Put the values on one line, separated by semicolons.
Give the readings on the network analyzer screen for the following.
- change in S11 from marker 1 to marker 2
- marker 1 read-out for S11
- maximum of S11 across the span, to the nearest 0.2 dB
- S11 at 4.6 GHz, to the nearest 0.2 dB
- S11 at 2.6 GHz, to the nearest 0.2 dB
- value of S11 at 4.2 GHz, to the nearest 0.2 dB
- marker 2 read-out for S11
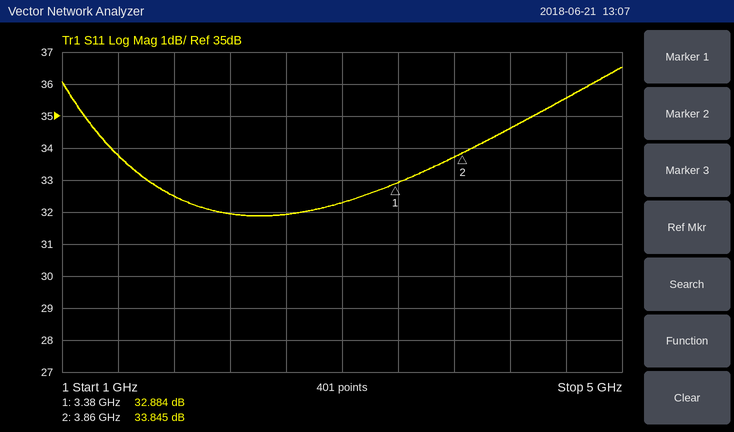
0.961 dB; 32.884 dB; 36.6 dB; 35.6 dB; 32.0 dB; 34.6 dB; 33.845 dB
